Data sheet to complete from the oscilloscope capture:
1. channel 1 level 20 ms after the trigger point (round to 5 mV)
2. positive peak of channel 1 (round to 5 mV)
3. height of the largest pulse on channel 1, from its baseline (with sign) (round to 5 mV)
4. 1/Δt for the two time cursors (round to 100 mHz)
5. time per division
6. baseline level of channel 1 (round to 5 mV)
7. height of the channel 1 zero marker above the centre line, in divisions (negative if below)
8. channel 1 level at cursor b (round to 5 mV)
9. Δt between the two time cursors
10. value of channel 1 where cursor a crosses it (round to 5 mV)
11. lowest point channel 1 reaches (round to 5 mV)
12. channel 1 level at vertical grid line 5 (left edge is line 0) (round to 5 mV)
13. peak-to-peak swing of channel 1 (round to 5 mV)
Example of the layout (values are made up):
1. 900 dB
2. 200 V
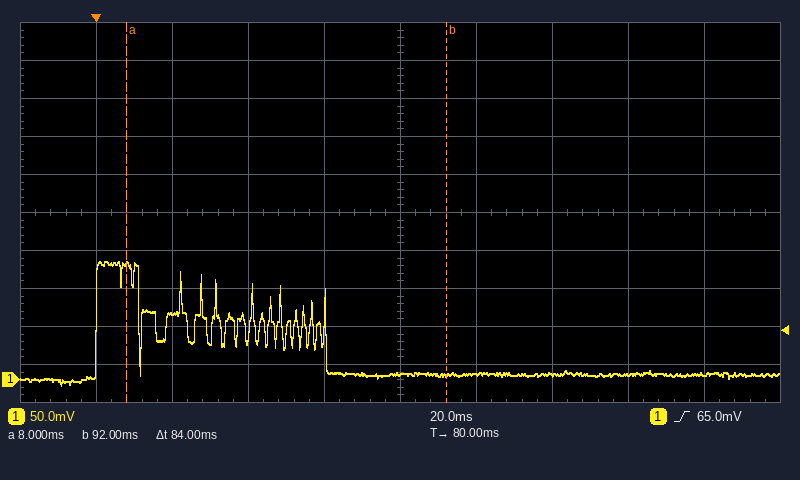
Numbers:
1. 85 mV
2. 155 mV
3. +150 mV
4. 11.9 Hz
5. 20 ms
6. 5 mV
7. -4.4 div
8. 5 mV
9. 84 ms
10. 150 mV
11. -10 mV
12. 10 mV
13. 165 mV
